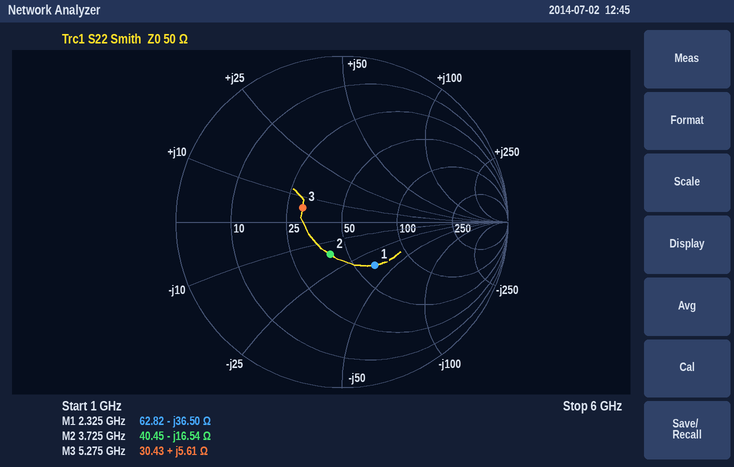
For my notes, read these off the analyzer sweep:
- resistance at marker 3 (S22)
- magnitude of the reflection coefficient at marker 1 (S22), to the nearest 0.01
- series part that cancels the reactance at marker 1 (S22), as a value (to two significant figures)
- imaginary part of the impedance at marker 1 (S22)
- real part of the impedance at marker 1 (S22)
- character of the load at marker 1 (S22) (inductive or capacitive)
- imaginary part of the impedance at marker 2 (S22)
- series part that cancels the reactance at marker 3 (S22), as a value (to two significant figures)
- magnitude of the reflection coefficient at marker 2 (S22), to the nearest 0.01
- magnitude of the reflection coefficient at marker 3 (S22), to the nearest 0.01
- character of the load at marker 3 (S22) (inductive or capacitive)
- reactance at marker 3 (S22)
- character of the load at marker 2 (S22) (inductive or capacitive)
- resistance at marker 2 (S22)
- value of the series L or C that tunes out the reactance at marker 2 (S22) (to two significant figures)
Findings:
30.43 Ω
0.33
2.5 nH
-36.50 Ω
62.82 Ω
capacitive
-16.54 Ω
5.4 pF
0.21
0.25
inductive
+5.61 Ω
capacitive
40.45 Ω
710 pH
